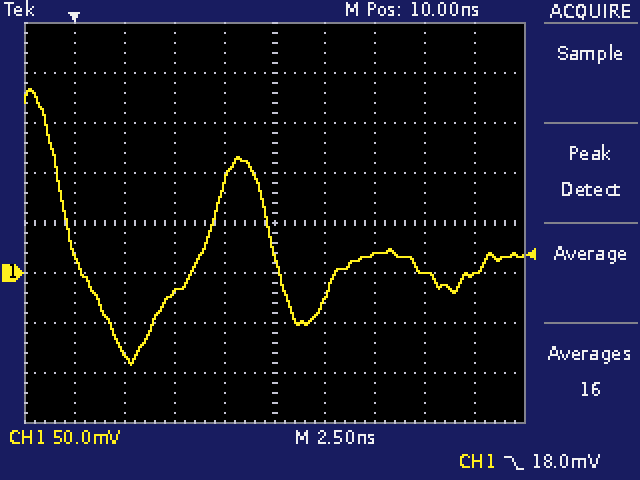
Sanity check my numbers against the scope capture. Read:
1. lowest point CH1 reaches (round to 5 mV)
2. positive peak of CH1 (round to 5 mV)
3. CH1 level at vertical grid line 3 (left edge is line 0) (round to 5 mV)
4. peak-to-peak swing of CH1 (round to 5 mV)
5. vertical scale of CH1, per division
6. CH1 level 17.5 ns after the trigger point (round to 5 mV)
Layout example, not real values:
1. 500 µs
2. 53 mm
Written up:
1. -90 mV
2. 185 mV
3. -20 mV
4. 275 mV
5. 50 mV
6. 0 mV
